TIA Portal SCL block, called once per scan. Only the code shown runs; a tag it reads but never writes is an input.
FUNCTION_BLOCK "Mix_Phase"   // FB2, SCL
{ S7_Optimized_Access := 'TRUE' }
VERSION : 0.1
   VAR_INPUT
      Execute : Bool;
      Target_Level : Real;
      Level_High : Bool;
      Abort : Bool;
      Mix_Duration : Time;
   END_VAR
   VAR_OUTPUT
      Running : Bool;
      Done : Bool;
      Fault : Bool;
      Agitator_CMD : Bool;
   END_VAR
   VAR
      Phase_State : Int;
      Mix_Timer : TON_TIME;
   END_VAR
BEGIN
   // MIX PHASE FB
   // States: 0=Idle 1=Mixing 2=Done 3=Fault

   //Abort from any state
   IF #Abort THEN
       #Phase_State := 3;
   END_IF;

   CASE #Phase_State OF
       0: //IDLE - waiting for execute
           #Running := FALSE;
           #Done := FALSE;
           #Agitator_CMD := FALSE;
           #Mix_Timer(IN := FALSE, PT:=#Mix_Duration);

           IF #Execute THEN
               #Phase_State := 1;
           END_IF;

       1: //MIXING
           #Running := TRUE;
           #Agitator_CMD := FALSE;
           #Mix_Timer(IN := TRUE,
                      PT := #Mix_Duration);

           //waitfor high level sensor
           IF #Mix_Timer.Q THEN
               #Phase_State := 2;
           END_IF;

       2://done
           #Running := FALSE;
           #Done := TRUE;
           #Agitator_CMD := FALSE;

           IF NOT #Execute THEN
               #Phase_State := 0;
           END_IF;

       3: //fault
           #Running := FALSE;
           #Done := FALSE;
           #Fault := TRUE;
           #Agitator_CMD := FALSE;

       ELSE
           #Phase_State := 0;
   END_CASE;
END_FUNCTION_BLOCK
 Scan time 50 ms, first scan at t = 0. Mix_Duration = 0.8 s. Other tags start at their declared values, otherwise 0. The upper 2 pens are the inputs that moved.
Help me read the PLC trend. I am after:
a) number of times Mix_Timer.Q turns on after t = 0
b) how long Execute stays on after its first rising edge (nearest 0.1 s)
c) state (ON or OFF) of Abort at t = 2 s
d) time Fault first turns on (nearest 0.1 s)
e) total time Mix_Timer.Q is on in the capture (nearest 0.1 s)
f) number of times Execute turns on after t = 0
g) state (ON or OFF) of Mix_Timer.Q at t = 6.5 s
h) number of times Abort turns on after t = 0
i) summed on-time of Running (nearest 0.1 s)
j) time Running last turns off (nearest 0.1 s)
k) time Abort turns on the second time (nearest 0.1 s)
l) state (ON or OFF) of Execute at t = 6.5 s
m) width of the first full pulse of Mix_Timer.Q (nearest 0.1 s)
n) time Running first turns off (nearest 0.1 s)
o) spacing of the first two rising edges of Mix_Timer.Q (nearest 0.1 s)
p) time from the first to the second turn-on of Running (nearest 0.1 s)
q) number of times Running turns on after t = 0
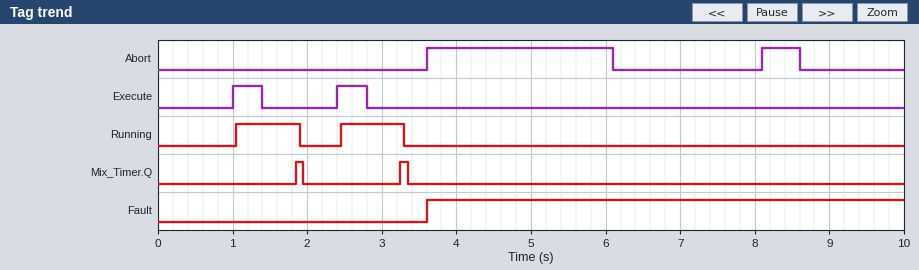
2
0.4 s
OFF
3.6 s
0.2 s
2
OFF
2
1.7 s
3.3 s
8.1 s
OFF
0.1 s
1.9 s
1.4 s
1.4 s
2
